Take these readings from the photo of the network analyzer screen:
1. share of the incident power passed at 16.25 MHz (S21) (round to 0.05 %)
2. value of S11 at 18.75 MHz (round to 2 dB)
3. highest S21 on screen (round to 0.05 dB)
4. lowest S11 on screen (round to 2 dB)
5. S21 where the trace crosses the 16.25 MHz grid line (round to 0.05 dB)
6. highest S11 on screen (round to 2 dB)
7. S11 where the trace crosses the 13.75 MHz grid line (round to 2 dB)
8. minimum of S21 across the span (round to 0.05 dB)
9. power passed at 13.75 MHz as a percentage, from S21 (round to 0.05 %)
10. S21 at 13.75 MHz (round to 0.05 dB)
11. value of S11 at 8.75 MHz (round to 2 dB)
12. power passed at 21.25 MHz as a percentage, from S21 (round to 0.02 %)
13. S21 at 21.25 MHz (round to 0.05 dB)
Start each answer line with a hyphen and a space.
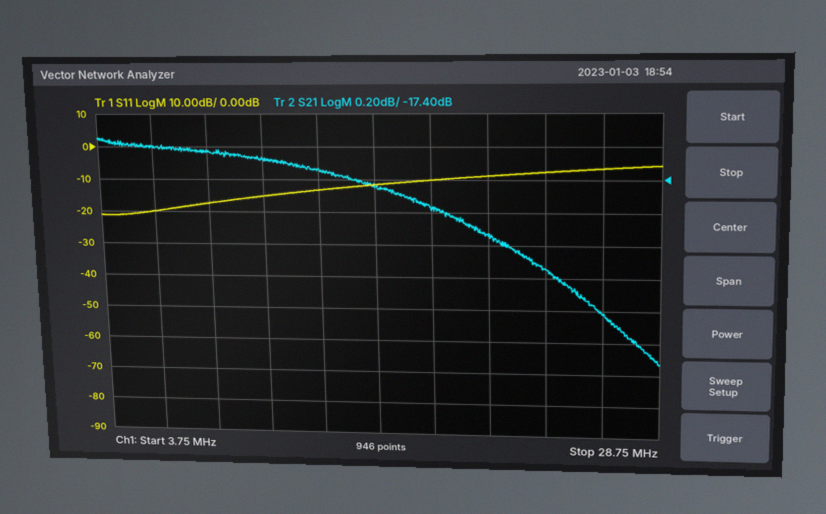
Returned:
- 1.80 %
- -10 dB
- -17.15 dB
- -22 dB
- -17.45 dB
- -6 dB
- -14 dB
- -18.55 dB
- 1.85 %
- -17.35 dB
- -18 dB
- 1.68 %
- -17.75 dB
